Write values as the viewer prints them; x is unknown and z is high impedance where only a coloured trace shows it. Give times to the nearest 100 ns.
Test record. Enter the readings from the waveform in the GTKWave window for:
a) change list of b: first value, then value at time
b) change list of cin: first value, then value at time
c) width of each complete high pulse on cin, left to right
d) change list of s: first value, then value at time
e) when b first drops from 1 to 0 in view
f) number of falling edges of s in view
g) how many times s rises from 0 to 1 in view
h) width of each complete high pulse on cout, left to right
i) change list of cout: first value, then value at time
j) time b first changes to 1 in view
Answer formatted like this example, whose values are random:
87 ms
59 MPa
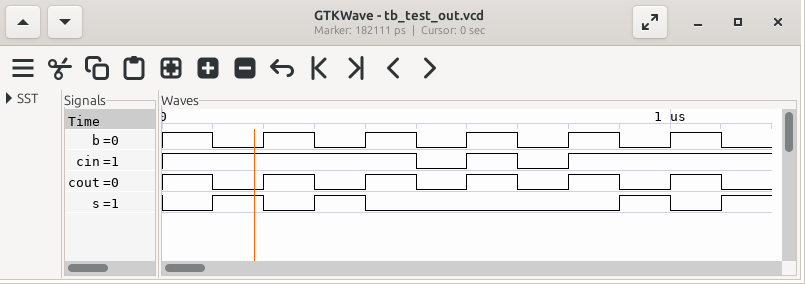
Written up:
1, 0 at 100 ns, 1 at 200 ns, 0 at 300 ns, 1 at 400 ns, 0 at 500 ns, 1 at 600 ns, 0 at 700 ns, 1 at 800 ns, 0 at 900 ns, 1 at 1000 ns, 0 at 1100 ns
1, 0 at 500 ns, 1 at 600 ns, 0 at 700 ns, 1 at 800 ns
100 ns
0, 1 at 100 ns, 0 at 200 ns, 1 at 300 ns, 0 at 400 ns, 1 at 900 ns, 0 at 1000 ns, 1 at 1100 ns
100 ns
3
4
100 ns, 100 ns, 100 ns, 100 ns, 100 ns
1, 0 at 100 ns, 1 at 200 ns, 0 at 300 ns, 1 at 400 ns, 0 at 500 ns, 1 at 600 ns, 0 at 700 ns, 1 at 800 ns, 0 at 900 ns, 1 at 1000 ns, 0 at 1100 ns
200 ns
